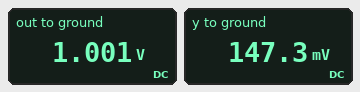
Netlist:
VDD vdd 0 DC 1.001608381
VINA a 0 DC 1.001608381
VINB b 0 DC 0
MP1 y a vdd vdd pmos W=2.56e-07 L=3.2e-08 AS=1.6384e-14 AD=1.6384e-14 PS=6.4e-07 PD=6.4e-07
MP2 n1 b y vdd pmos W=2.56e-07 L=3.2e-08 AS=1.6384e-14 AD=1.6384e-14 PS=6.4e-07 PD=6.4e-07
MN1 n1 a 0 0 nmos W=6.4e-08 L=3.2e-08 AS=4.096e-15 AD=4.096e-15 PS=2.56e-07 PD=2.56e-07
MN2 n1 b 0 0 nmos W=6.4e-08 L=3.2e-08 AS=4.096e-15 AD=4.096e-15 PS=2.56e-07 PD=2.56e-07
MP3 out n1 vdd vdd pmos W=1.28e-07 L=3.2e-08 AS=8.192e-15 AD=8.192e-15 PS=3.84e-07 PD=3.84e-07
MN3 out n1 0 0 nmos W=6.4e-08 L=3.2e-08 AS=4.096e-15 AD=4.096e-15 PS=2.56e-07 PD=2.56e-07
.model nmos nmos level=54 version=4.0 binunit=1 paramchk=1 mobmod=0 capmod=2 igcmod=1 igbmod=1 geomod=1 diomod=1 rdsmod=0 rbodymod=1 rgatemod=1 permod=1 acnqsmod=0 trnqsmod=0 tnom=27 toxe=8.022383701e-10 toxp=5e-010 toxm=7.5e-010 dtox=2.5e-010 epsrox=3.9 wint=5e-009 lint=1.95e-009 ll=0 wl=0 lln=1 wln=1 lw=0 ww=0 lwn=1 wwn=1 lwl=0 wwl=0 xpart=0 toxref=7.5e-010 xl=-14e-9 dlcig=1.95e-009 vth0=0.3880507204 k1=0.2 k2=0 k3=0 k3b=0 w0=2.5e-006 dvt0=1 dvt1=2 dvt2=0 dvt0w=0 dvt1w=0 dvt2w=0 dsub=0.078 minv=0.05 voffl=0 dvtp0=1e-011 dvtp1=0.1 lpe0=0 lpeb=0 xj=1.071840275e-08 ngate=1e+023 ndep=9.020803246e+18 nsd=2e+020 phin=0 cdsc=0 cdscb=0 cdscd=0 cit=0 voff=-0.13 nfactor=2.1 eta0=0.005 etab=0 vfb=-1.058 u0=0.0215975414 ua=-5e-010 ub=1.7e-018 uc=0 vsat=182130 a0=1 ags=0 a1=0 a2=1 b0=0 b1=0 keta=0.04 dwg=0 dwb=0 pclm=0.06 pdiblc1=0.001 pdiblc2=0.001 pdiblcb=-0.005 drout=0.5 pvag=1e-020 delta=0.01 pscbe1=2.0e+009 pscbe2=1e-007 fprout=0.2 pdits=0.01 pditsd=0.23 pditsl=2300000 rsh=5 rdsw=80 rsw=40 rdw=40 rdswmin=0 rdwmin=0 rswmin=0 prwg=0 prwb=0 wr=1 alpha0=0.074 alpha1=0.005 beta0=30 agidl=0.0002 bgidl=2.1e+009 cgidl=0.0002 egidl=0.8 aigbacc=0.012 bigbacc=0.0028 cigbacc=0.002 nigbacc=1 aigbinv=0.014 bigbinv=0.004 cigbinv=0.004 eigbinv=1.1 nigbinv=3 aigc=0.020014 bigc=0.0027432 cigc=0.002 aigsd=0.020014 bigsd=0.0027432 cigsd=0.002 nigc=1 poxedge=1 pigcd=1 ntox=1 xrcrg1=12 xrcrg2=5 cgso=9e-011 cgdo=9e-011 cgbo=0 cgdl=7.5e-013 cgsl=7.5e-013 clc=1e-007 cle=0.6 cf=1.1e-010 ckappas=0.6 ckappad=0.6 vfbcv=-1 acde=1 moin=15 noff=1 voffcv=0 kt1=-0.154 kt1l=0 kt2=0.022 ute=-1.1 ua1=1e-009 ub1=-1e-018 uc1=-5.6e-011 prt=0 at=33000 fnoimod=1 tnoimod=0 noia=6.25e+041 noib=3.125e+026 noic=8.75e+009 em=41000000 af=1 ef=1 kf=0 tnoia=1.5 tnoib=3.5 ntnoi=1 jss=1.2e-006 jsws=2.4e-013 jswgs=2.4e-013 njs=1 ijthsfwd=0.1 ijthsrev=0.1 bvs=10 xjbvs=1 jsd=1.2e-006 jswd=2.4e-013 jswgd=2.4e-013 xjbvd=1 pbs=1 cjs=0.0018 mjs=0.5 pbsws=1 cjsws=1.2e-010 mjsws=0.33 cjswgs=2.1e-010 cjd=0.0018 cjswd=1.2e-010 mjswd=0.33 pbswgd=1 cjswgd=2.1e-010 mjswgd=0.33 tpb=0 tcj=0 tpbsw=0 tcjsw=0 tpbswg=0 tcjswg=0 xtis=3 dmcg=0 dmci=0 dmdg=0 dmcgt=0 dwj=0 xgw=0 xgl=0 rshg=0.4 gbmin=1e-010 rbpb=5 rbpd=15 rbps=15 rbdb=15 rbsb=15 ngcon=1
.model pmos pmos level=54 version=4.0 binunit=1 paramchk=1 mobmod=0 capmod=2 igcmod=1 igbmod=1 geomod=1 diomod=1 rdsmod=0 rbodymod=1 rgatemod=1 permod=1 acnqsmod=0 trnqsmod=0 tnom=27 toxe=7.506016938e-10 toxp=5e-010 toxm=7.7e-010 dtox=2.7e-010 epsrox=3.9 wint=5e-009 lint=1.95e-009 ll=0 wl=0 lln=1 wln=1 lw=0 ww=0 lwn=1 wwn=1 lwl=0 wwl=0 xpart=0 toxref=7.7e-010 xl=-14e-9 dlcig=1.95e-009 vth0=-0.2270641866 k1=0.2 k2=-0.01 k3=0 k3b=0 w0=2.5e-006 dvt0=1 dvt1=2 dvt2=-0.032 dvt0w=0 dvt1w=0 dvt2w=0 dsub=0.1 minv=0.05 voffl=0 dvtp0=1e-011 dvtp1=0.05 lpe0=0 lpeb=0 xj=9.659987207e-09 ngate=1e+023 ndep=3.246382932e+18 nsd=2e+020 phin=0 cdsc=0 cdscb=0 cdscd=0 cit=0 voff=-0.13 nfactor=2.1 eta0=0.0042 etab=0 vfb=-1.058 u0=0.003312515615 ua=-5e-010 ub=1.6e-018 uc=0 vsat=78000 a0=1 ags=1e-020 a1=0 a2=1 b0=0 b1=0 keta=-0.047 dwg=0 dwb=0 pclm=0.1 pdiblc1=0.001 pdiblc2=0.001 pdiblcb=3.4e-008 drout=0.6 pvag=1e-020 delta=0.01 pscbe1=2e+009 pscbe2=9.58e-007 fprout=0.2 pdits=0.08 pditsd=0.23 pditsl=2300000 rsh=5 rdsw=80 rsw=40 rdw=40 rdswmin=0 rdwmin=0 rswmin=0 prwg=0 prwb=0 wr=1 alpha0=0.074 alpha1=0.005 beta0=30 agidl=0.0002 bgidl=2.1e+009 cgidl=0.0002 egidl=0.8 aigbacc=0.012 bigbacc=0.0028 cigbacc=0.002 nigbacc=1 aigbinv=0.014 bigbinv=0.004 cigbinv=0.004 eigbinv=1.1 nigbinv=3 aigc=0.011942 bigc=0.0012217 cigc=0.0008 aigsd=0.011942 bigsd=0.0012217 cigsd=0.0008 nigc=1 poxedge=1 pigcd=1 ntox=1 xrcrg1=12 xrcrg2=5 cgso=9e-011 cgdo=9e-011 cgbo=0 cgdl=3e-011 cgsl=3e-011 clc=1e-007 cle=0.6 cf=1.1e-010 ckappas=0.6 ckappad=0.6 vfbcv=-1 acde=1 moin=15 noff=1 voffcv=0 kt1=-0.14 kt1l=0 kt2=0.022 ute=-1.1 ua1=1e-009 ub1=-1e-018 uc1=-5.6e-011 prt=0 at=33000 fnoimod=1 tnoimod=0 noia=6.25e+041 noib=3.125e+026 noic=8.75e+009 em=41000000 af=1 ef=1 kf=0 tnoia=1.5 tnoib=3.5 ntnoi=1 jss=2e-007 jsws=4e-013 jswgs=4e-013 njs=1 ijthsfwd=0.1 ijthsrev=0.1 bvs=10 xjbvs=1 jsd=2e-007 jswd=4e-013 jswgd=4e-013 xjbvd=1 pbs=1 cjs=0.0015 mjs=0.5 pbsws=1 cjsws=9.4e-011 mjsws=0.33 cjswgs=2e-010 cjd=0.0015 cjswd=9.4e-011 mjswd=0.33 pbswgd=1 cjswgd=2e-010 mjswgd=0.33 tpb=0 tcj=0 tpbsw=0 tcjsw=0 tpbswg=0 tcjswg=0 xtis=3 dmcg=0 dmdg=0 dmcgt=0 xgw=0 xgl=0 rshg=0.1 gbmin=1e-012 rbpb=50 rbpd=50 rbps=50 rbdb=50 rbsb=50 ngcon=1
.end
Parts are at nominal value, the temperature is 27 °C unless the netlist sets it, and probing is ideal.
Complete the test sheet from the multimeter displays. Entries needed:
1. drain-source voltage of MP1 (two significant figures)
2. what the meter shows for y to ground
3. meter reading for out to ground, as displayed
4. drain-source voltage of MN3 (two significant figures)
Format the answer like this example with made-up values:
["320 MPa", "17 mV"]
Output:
["-850 mV", "147.3 mV", "1.001 V", "1.0 V"]
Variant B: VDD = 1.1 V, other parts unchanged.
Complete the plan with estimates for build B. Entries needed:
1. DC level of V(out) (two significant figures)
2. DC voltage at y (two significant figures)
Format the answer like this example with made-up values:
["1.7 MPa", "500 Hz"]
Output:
["1.1 V", "230 mV"]
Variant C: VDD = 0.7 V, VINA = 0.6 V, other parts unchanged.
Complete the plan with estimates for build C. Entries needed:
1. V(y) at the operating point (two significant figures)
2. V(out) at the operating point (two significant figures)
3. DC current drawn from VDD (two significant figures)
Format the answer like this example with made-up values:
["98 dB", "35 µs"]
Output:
["180 mV", "700 mV", "790 nA"]
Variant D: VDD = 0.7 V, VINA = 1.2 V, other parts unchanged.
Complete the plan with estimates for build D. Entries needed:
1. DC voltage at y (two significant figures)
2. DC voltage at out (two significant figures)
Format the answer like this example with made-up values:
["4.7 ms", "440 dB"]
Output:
["93 mV", "700 mV"]
